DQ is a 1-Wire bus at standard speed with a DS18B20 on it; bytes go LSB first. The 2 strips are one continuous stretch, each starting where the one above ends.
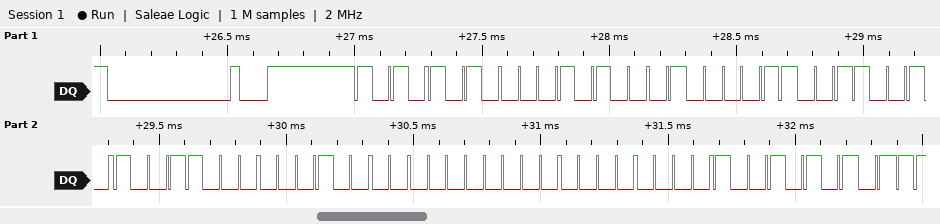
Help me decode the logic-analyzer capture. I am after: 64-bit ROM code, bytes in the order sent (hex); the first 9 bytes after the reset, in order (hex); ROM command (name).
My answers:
28 C2 4C 19 08 00 00 A9
55 28 C2 4C 19 08 00 00 A9
Match ROM
